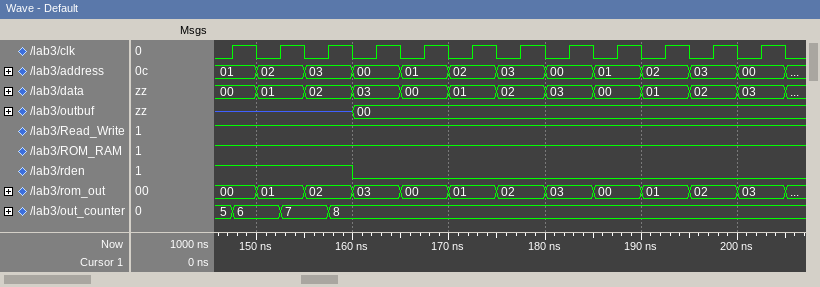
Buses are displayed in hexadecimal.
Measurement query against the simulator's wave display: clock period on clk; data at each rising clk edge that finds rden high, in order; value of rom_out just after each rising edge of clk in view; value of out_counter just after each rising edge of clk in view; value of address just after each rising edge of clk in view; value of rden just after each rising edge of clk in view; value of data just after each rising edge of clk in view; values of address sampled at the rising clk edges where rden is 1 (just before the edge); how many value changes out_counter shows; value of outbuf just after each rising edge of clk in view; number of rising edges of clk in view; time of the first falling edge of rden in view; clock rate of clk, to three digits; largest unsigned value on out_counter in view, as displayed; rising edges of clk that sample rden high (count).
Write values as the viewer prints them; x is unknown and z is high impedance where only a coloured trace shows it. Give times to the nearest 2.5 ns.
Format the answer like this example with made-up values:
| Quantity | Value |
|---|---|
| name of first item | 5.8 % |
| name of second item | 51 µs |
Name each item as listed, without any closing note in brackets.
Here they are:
| Quantity | Value |
|---|---|
| clock period on clk | 5 ns |
| data at each rising clk edge that finds rden high, in order | 00, 01, 02 |
| value of rom_out just after each rising edge of clk in view | 00, 01, 02, 03, 00, 01, 02, 03, 00, 01, 02, 03 |
| value of out_counter just after each rising edge of clk in view | 6, 7, 8, 8, 8, 8, 8, 8, 8, 8, 8, 8 |
| value of address just after each rising edge of clk in view | 01, 02, 03, 00, 01, 02, 03, 00, 01, 02, 03, 00 |
| value of rden just after each rising edge of clk in view | 1 1 1 0 0 0 0 0 0 0 0 0 |
| value of data just after each rising edge of clk in view | 00, 01, 02, 03, 00, 01, 02, 03, 00, 01, 02, 03 |
| values of address sampled at the rising clk edges where rden is 1 | 01, 02, 03 |
| how many value changes out_counter shows | 3 |
| value of outbuf just after each rising edge of clk in view | z, z, z, 00, 00, 00, 00, 00, 00, 00, 00, 00 |
| number of rising edges of clk in view | 12 |
| time of the first falling edge of rden in view | 160 ns |
| clock rate of clk, to three digits | 200 MHz |
| largest unsigned value on out_counter in view, as displayed | 8 |
| rising edges of clk that sample rden high | 3 |
